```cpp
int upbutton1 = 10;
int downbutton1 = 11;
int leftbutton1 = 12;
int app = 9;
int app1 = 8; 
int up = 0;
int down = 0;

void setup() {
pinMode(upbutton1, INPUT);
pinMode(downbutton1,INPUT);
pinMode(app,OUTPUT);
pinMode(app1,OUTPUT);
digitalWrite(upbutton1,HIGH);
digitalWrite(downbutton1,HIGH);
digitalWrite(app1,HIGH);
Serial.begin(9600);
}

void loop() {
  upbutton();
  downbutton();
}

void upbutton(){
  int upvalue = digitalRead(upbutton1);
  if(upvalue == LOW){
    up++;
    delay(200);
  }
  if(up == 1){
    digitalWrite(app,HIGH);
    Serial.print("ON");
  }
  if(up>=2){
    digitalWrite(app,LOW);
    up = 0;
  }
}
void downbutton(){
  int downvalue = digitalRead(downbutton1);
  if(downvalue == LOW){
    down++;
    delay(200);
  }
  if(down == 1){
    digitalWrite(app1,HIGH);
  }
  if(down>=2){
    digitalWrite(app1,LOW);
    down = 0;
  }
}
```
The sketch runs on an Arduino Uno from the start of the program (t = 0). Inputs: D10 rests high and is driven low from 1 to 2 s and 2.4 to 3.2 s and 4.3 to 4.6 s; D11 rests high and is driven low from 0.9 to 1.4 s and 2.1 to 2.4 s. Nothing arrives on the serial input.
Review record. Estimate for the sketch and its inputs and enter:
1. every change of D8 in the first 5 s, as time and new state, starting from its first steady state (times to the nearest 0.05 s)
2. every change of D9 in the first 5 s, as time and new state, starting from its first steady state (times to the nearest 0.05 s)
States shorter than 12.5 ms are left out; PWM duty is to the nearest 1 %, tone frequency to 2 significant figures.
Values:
0 s high; 1.5 s low; 2.3 s high; 2.5 s low
0 s low; 1.3 s high; 1.7 s low; 1.9 s high; 2.1 s low; 2.7 s high; 2.9 s low; 3.1 s high; 3.3 s low; 4.5 s high; 4.7 s low
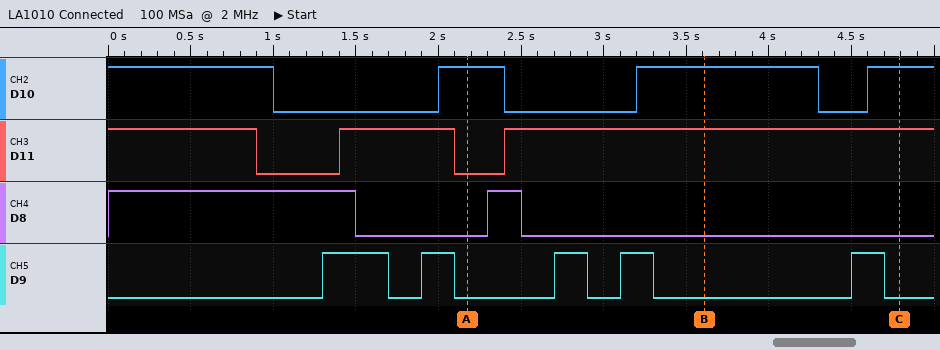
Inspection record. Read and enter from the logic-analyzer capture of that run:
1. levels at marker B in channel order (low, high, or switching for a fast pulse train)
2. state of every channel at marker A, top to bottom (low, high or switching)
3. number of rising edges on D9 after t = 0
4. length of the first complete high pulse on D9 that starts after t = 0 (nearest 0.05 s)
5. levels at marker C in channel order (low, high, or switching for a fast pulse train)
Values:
D10 high, D11 high, D8 low, D9 low
D10 high, D11 low, D8 low, D9 low
5
0.40 s
D10 high, D11 high, D8 low, D9 low
